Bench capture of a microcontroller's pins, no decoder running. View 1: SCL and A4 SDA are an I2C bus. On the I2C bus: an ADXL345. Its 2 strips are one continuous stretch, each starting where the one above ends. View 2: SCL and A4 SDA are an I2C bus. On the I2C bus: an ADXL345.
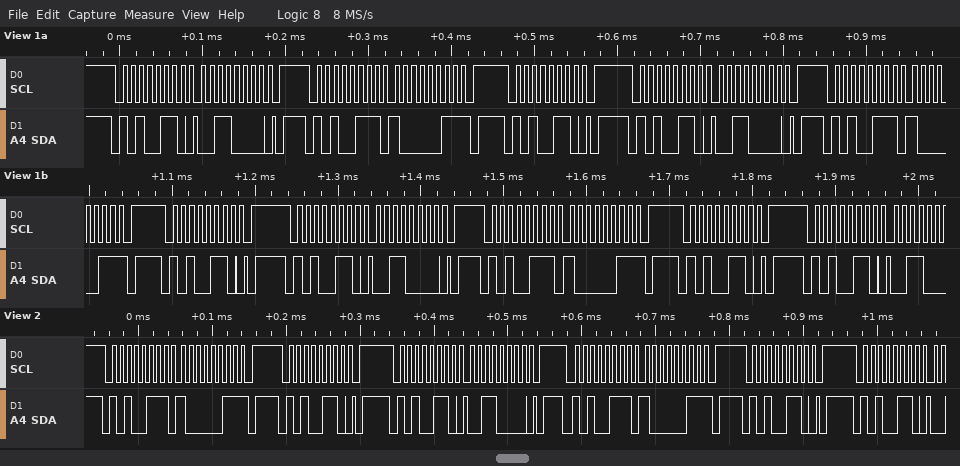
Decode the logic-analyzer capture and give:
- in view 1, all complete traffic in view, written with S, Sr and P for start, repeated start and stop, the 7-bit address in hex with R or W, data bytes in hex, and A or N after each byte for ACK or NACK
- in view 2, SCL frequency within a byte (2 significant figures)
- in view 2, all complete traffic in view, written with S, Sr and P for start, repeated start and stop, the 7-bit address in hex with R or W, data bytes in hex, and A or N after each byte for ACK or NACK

S 53W A 30 A P S 53R A 83 N P S 53W A P S 53W A 30 A P S 53R A 83 N P S 53W A P S 53W A 30 A P S 53R A 83 N P S 53W A P S 53W A
100 kHz
S 53R A 83 N P S 53W A P S 53W A 30 A P S 53R A 83 N P S 53W A P S 53W A
